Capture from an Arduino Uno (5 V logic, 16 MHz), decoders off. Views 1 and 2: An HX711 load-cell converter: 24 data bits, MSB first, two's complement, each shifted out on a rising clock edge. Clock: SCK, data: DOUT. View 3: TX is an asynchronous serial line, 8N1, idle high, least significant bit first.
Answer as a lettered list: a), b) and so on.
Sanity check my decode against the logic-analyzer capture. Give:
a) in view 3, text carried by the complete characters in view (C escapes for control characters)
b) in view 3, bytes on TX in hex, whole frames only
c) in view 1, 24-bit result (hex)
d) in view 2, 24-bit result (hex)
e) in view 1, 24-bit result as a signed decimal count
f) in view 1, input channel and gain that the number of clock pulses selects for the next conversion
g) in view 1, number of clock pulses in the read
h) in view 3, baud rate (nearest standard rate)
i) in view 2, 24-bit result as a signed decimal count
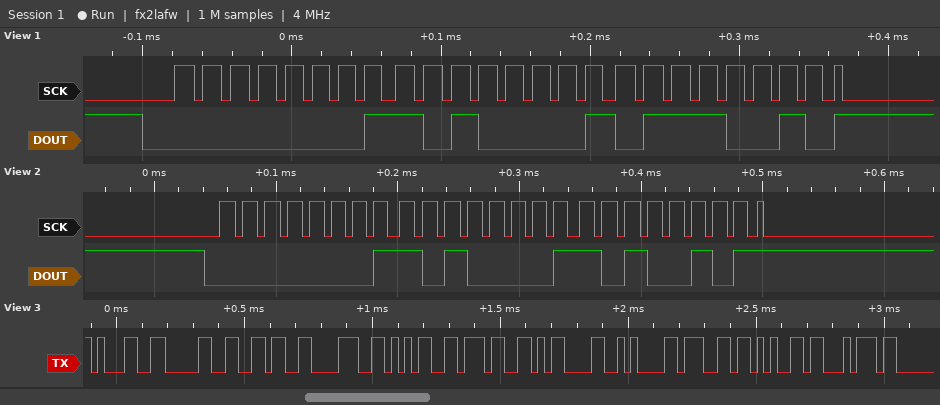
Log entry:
a) "106857\r\nget"
b) 31 30 36 38 35 37 0D 0A 67 65 74
c) 0x01A172
d) 0x01A1A5
e) 106866
f) channel A, gain 128
g) 25
h) 38400 baud
i) 106917
